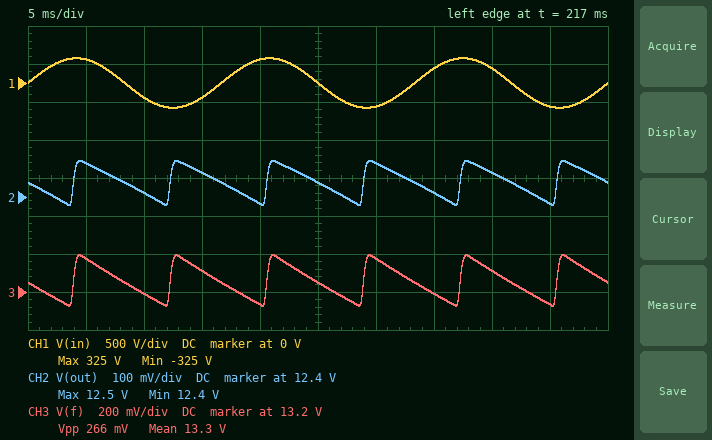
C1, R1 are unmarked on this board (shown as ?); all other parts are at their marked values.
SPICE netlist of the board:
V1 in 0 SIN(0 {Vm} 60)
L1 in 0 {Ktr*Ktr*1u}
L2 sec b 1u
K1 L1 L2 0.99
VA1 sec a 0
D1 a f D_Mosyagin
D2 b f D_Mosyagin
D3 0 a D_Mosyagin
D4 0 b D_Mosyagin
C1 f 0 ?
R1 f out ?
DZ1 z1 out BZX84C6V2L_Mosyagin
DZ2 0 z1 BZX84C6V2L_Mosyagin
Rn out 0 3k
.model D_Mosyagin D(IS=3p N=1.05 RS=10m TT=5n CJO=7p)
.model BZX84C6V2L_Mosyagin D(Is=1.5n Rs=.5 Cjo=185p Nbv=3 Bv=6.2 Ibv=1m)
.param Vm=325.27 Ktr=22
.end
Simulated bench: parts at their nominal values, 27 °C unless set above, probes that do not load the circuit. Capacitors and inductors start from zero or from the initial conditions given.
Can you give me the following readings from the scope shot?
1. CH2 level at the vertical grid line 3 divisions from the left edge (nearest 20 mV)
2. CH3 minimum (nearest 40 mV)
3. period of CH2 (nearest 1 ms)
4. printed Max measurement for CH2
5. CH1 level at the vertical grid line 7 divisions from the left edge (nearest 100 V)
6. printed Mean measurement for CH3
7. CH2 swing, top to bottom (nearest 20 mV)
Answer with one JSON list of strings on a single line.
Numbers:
["12.46 V", "13.12 V", "8 ms", "12.5 V", "200 V", "13.3 V", "120 mV"]
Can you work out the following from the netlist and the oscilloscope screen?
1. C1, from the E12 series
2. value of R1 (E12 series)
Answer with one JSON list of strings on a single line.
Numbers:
["150 µF", "150 Ω"]
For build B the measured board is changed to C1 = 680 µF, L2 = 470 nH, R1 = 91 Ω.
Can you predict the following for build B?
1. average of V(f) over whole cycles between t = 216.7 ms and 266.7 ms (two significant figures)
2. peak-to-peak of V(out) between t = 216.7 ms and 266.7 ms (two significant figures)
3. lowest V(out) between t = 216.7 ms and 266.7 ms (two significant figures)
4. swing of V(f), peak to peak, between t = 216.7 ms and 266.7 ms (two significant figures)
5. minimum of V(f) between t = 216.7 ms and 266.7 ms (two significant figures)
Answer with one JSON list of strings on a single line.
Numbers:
["8.8 V", "29 mV", "8.5 V", "30 mV", "8.7 V"]
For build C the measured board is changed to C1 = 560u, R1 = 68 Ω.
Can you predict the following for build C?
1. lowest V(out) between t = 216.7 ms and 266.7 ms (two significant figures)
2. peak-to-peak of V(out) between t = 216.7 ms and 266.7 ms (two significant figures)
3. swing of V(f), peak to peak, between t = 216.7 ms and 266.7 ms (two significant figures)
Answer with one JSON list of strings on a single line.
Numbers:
["13 V", "39 mV", "120 mV"]
